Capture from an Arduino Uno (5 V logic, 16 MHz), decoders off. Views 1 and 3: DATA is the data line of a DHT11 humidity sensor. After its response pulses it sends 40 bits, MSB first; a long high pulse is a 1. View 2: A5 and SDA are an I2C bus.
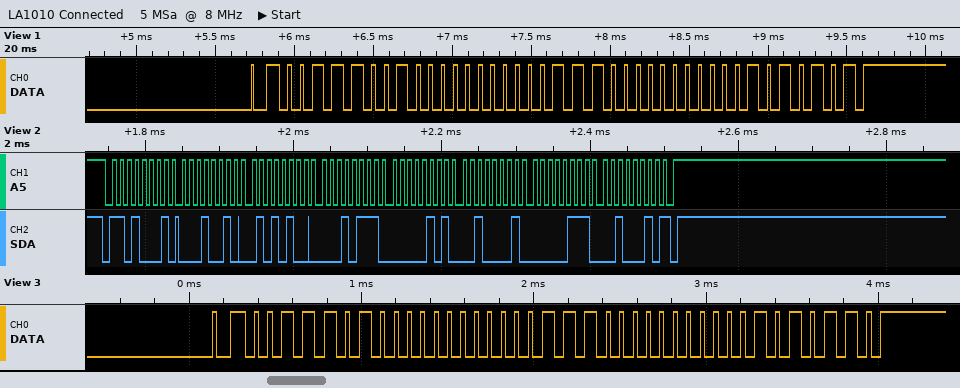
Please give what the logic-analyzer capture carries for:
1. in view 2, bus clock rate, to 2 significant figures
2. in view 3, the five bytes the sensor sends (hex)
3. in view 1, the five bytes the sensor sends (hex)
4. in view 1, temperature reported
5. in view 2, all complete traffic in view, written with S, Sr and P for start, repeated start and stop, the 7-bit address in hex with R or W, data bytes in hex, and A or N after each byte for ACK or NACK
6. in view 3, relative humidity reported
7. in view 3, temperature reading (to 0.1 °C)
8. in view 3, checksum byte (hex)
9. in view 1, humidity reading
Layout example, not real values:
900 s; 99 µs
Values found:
100 kHz; 3A 00 1C 00 56; 39 00 1C 00 55; 28.0 °C; S 68R A 12 A 54 A 17 A 05 A 21 A 07 A 22 N P; 58 %; 28.0 °C; 0x56; 57 %
